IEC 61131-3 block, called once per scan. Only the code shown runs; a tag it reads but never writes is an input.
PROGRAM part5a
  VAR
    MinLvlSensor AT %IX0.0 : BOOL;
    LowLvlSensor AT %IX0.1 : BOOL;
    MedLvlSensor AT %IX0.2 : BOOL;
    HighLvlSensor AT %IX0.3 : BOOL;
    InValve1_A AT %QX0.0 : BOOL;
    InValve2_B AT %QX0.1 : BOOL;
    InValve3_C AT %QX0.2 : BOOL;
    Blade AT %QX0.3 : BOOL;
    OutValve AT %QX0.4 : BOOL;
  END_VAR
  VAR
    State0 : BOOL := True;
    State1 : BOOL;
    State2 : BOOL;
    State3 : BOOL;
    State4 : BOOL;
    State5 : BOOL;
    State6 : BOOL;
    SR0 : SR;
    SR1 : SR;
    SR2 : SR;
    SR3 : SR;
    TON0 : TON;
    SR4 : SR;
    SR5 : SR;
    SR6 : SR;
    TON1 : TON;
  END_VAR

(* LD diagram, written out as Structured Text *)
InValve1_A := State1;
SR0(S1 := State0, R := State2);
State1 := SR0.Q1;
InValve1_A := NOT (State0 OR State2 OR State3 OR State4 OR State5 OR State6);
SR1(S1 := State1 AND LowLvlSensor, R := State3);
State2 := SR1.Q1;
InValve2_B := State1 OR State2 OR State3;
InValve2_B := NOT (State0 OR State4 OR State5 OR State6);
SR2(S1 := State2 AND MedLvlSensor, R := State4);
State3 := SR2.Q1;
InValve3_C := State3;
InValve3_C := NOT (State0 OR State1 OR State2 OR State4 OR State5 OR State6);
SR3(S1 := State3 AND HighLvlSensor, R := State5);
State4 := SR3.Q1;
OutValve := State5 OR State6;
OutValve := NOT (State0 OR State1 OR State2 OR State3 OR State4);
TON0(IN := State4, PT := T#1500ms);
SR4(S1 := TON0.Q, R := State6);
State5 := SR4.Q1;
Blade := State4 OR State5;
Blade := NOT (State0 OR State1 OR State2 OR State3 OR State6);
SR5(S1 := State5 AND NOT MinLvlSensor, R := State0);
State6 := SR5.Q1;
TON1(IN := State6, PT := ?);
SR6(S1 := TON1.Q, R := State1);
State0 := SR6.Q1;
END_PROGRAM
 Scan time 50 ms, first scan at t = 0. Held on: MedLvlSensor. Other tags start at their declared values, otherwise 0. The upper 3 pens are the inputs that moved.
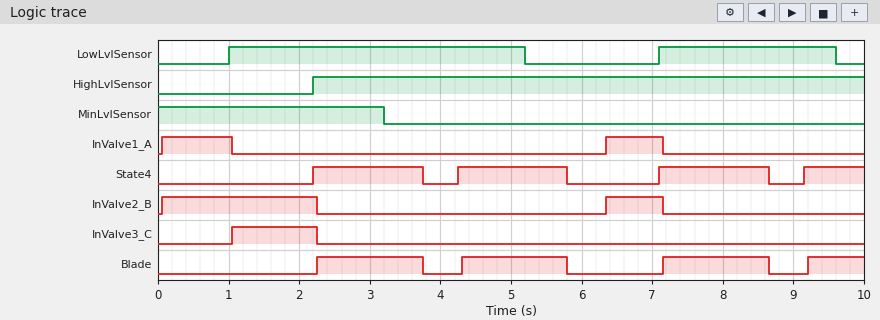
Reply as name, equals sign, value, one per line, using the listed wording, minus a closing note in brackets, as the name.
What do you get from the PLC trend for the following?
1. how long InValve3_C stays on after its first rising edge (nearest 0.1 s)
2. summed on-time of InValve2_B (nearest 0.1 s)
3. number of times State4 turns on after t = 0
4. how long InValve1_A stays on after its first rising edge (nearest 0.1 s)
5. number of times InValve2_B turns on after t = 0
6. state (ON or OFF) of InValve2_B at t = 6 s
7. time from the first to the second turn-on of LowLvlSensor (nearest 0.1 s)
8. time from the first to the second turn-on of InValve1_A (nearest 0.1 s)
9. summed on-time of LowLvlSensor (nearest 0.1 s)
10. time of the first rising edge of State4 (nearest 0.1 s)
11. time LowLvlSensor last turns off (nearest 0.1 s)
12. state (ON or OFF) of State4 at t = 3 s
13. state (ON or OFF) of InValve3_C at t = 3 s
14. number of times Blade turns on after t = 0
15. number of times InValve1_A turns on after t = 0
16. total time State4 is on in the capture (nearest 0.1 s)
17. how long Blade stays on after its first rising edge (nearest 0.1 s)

how long InValve3_C stays on after its first rising edge = 1.2 s
summed on-time of InValve2_B = 3.0 s
number of times State4 turns on after t = 0 = 4
how long InValve1_A stays on after its first rising edge = 1.0 s
number of times InValve2_B turns on after t = 0 = 2
state (ON or OFF) of InValve2_B at t = 6 s = OFF
time from the first to the second turn-on of LowLvlSensor = 6.1 s
time from the first to the second turn-on of InValve1_A = 6.3 s
summed on-time of LowLvlSensor = 6.7 s
time of the first rising edge of State4 = 2.2 s
time LowLvlSensor last turns off = 9.6 s
state (ON or OFF) of State4 at t = 3 s = ON
state (ON or OFF) of InValve3_C at t = 3 s = OFF
number of times Blade turns on after t = 0 = 4
number of times InValve1_A turns on after t = 0 = 2
total time State4 is on in the capture = 5.5 s
how long Blade stays on after its first rising edge = 1.5 s
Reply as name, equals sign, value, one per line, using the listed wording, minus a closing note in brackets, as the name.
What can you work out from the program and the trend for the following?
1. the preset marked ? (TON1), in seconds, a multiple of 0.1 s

the preset marked ? (TON1), in seconds, a multiple of 0.1 s = 0.5 s
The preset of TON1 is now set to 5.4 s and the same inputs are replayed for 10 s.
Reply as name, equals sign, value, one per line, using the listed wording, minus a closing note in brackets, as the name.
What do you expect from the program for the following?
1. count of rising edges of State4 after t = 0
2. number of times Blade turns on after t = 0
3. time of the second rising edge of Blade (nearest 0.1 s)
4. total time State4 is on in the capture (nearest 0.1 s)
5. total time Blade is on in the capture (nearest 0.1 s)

count of rising edges of State4 after t = 0 = 2
number of times Blade turns on after t = 0 = 2
time of the second rising edge of Blade = 9.2 s
total time State4 is on in the capture = 2.4 s
total time Blade is on in the capture = 2.3 s
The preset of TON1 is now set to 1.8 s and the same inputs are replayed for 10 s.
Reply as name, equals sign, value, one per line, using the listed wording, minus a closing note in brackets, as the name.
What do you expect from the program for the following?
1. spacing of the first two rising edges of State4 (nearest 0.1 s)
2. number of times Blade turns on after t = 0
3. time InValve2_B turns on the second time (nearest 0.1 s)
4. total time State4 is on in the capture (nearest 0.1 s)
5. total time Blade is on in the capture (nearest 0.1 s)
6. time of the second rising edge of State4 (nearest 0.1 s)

spacing of the first two rising edges of State4 = 4.9 s
number of times Blade turns on after t = 0 = 2
time InValve2_B turns on the second time = 5.6 s
total time State4 is on in the capture = 3.1 s
total time Blade is on in the capture = 3.0 s
time of the second rising edge of State4 = 7.1 s
